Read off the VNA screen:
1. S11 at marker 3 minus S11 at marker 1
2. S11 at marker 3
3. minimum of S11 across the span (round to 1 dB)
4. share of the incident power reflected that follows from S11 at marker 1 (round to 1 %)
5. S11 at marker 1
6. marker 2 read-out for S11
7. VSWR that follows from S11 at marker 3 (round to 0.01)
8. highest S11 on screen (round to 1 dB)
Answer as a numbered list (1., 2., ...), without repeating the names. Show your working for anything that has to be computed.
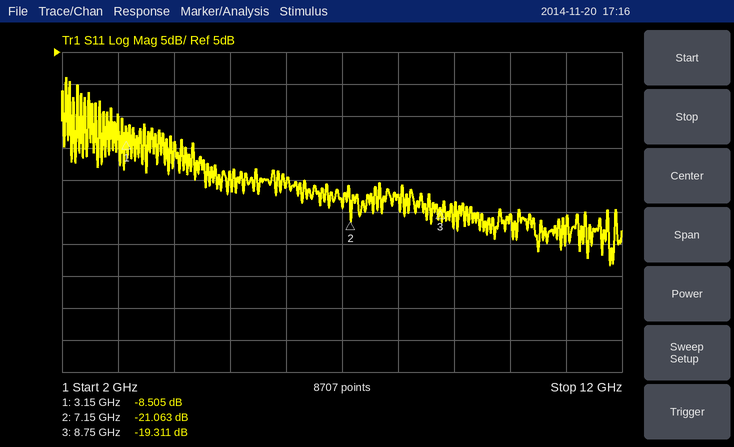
1. -19.311 − (-8.505) = -10.806 dB
2. -19.311 dB
3. -28 dB
4. 10^(-8.505/10) ≈ 14 %
5. -8.505 dB
6. -21.063 dB
7. (1 + 0.1083)/(1 − 0.1083) ≈ 1.24
8. 1 dB
